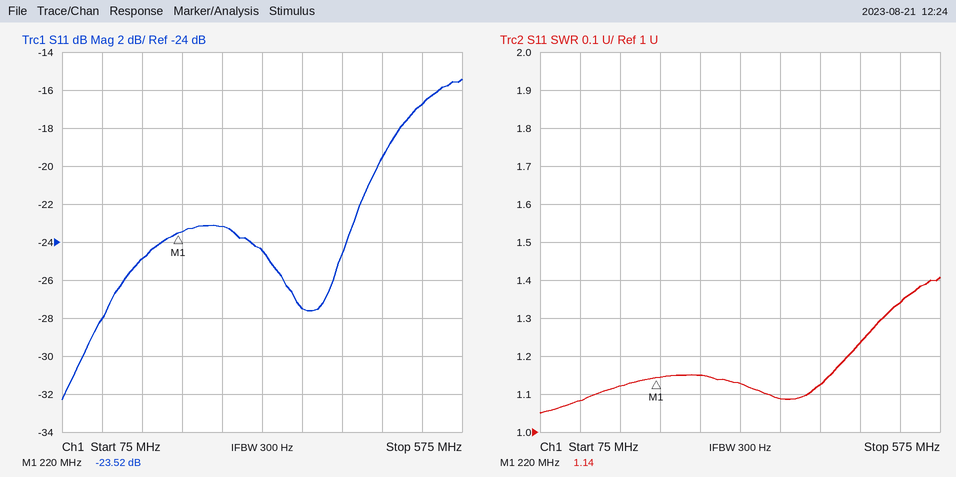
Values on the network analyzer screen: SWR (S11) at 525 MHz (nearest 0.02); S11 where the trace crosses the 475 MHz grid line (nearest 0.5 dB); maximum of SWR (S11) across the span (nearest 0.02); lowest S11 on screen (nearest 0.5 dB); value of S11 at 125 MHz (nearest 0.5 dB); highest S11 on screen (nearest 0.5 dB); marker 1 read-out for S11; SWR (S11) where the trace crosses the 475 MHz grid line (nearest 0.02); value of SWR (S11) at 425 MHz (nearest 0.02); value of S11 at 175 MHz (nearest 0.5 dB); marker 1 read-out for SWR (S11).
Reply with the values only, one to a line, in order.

1.34
-19.5 dB
1.40
-32.5 dB
-28.0 dB
-15.5 dB
-23.52 dB
1.24
1.12
-25.0 dB
1.14
